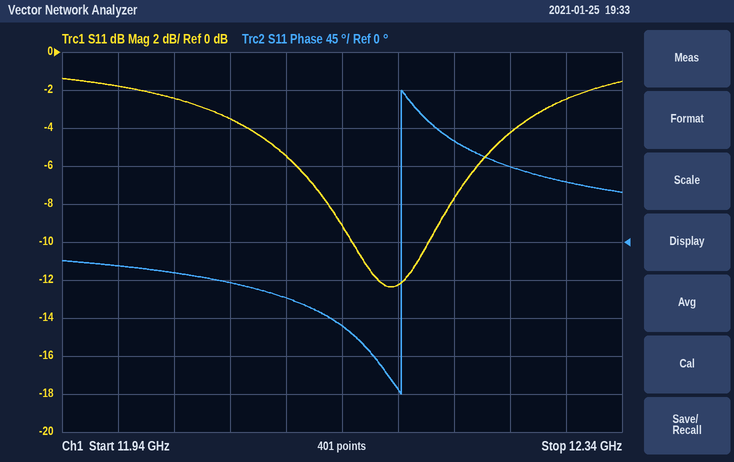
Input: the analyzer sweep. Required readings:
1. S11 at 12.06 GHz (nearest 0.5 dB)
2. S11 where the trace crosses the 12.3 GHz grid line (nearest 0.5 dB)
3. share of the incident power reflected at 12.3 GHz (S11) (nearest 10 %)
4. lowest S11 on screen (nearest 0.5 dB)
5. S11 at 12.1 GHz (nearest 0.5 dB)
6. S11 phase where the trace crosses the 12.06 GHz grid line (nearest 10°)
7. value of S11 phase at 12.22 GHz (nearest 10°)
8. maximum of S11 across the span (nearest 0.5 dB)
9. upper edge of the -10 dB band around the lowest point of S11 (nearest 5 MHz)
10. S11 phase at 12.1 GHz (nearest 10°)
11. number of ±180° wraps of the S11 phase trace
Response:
-3.5 dB
-2.5 dB
60 %
-12.5 dB
-5.5 dB
-50°
120°
-1.5 dB
12.200 GHz
-70°
1
